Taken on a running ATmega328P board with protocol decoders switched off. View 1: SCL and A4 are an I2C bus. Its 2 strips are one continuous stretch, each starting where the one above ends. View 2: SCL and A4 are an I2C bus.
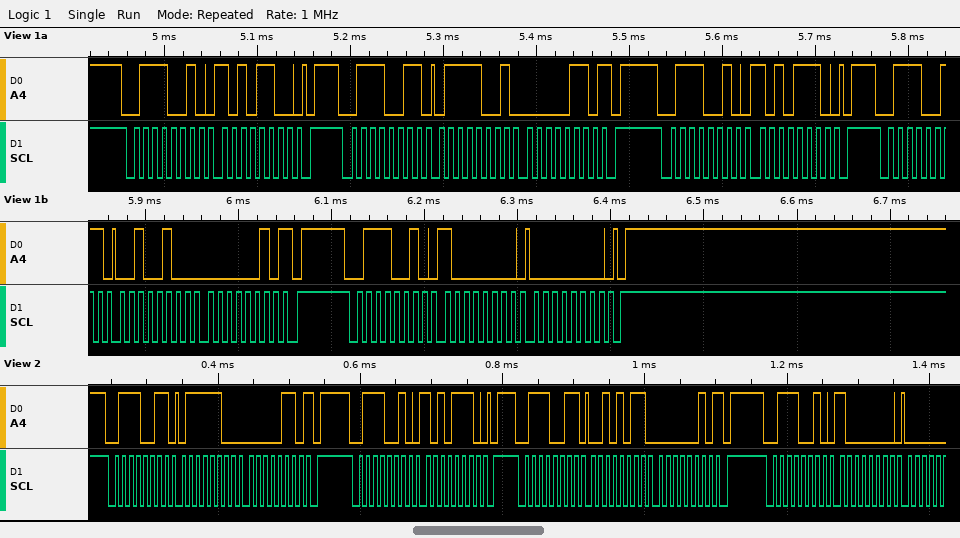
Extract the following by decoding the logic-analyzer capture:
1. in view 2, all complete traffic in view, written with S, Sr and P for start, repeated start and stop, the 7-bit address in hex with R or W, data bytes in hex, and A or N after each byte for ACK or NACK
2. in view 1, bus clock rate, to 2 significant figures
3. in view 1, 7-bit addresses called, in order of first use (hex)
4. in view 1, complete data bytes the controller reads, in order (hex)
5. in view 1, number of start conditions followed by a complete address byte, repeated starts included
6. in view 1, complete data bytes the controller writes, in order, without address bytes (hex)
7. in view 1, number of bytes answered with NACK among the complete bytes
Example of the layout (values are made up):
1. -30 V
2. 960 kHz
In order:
1. S 39R A 7C A 06 N P S 39W A AE A P S 39R A 2B A 02 N P S 39W A 80 A
2. 100 kHz
3. 0x39
4. 79 06 24 02
5. 5
6. AC AE 80 00
7. 2
